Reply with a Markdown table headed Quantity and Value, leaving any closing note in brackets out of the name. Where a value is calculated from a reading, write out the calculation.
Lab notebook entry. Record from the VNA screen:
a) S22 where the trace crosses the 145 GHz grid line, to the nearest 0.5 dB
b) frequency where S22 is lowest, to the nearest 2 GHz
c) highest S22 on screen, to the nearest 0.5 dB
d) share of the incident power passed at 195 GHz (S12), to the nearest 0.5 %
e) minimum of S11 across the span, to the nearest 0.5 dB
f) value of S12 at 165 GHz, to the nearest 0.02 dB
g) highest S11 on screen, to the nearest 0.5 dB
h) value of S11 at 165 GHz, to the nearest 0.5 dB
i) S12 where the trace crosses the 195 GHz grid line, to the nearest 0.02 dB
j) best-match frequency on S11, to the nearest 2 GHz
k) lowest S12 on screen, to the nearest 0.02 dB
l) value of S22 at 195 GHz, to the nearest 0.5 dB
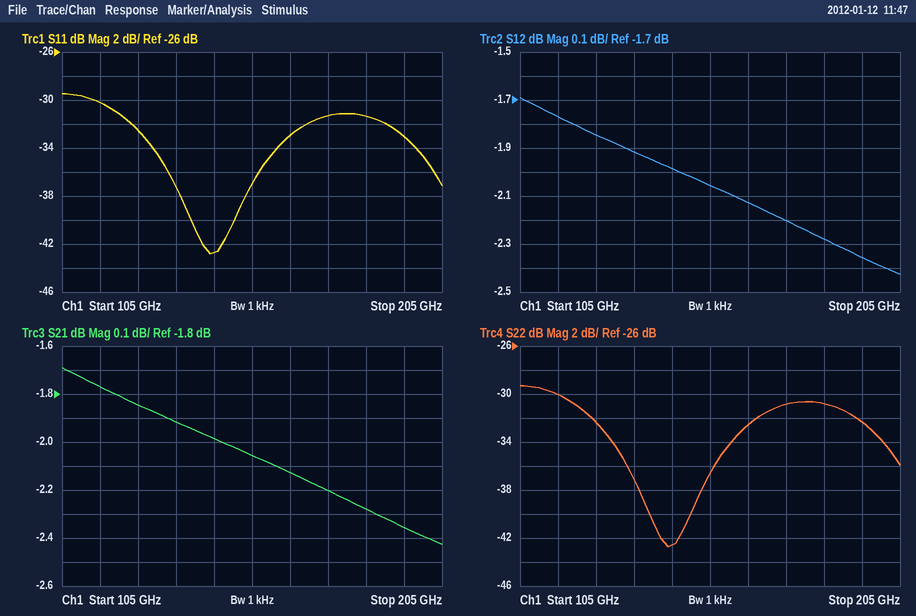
| Quantity | Value |
|---|---|
| S22 where the trace crosses the 145 GHz grid line, to the nearest 0.5 dB | -42.5 dB |
| frequency where S22 is lowest, to the nearest 2 GHz | 144 GHz |
| highest S22 on screen, to the nearest 0.5 dB | -29.5 dB |
| share of the incident power passed at 195 GHz (S12), to the nearest 0.5 % | 10^(-2.36/10) ≈ 58.1 %, so 58.0 % to the nearest 0.5 % |
| minimum of S11 across the span, to the nearest 0.5 dB | -43.0 dB |
| value of S12 at 165 GHz, to the nearest 0.02 dB | -2.12 dB |
| highest S11 on screen, to the nearest 0.5 dB | -29.5 dB |
| value of S11 at 165 GHz, to the nearest 0.5 dB | -33.0 dB |
| S12 where the trace crosses the 195 GHz grid line, to the nearest 0.02 dB | -2.36 dB |
| best-match frequency on S11, to the nearest 2 GHz | 144 GHz |
| lowest S12 on screen, to the nearest 0.02 dB | -2.42 dB |
| value of S22 at 195 GHz, to the nearest 0.5 dB | -32.5 dB |
